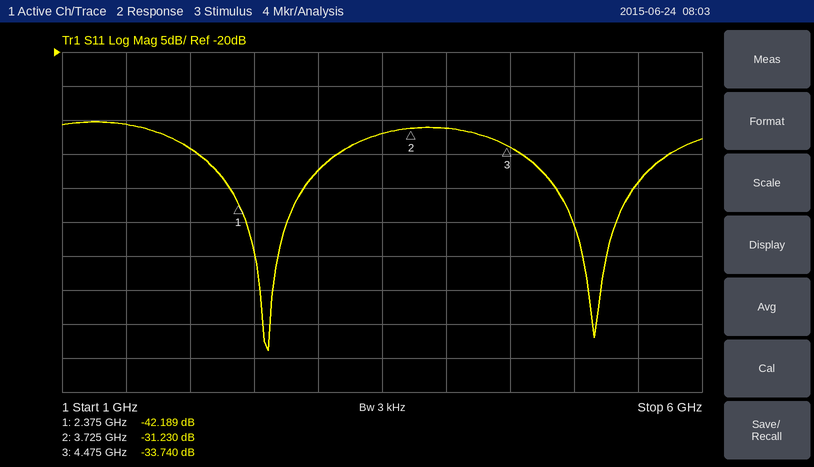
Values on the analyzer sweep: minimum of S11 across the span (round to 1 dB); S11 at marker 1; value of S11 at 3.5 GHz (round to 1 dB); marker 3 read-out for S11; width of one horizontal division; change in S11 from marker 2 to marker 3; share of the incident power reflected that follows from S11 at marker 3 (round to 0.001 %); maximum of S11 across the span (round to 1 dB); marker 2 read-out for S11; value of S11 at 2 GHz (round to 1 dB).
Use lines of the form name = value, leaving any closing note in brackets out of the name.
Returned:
minimum of S11 across the span = -64 dB
S11 at marker 1 = -42.189 dB
value of S11 at 3.5 GHz = -32 dB
marker 3 read-out for S11 = -33.740 dB
width of one horizontal division = 500 MHz
change in S11 from marker 2 to marker 3 = -2.510 dB
share of the incident power reflected that follows from S11 at marker 3 = 0.042 %
maximum of S11 across the span = -30 dB
marker 2 read-out for S11 = -31.230 dB
value of S11 at 2 GHz = -34 dB
